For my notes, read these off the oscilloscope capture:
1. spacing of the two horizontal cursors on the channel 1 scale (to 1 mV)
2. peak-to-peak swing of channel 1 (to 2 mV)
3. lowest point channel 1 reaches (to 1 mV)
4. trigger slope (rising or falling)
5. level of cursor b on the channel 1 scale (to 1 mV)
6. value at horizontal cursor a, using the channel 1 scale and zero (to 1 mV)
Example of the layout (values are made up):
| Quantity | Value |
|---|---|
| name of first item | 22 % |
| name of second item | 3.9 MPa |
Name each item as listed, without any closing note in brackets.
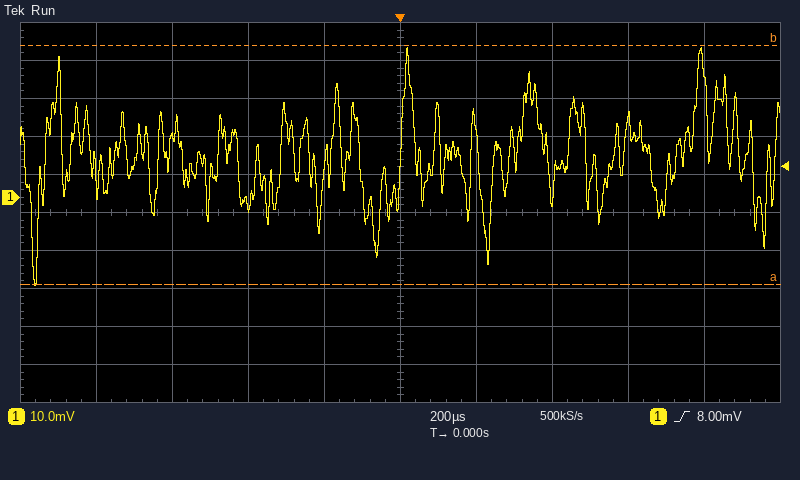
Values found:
| Quantity | Value |
|---|---|
| spacing of the two horizontal cursors on the channel 1 scale | 63 mV |
| peak-to-peak swing of channel 1 | 62 mV |
| lowest point channel 1 reaches | -23 mV |
| trigger slope | rising |
| level of cursor b on the channel 1 scale | 40 mV |
| value at horizontal cursor a, using the channel 1 scale and zero | -23 mV |
